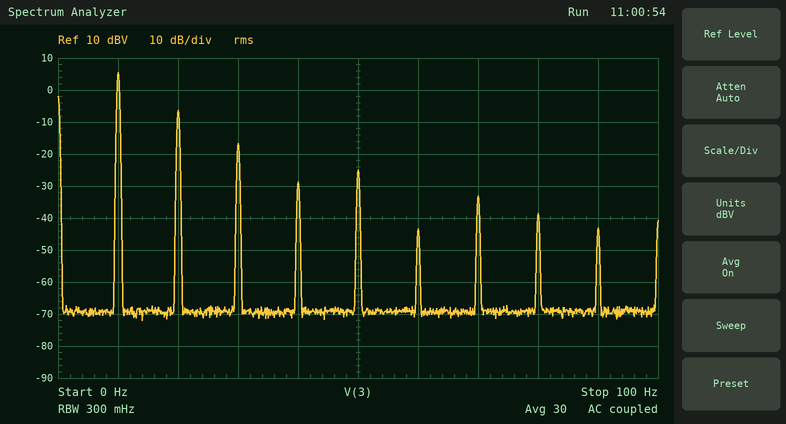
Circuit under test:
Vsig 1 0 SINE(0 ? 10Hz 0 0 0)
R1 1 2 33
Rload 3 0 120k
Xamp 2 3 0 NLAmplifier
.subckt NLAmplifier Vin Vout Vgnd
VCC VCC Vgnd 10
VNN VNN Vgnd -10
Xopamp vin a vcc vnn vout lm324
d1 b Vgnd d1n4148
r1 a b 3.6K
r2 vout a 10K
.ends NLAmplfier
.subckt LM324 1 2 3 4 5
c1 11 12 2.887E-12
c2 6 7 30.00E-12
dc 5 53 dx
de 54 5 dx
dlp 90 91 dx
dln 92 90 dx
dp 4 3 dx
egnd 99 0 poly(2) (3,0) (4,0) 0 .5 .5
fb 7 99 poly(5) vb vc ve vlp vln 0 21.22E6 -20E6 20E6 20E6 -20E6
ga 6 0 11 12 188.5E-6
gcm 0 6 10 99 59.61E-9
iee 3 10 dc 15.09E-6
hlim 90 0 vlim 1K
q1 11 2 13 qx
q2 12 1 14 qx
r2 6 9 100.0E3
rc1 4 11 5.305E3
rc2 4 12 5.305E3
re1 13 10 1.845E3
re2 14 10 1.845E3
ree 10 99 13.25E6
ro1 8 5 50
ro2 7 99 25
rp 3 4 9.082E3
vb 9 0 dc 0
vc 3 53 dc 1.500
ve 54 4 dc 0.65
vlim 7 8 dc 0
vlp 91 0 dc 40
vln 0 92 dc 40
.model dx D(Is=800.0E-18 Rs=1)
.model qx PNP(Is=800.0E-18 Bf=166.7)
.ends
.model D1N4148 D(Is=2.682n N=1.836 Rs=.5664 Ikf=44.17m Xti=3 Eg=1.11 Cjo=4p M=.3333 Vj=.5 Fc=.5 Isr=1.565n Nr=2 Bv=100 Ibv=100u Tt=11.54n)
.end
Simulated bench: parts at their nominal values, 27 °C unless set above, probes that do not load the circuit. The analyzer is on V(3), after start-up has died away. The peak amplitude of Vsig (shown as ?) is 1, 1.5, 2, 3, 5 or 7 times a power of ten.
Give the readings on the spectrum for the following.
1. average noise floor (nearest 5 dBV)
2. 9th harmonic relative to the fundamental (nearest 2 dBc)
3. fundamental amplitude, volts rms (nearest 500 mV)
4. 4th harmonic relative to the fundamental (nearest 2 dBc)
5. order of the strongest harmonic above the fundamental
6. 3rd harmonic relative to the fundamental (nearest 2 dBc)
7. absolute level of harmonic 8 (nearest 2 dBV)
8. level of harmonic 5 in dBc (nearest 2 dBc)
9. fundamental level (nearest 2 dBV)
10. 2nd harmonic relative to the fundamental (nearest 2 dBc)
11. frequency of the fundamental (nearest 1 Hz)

-70 dBV
-48 dBc
2.0 V
-34 dBc
2
-22 dBc
-38 dBV
-30 dBc
6 dBV
-12 dBc
10 Hz
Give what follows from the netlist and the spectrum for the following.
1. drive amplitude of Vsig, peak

1.5 V
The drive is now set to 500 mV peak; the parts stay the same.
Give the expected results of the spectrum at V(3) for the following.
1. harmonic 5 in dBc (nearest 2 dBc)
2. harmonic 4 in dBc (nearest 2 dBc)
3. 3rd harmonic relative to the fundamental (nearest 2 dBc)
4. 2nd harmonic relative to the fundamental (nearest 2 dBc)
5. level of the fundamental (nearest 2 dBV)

-40 dBc
-30 dBc
-24 dBc
-20 dBc
-8 dBV
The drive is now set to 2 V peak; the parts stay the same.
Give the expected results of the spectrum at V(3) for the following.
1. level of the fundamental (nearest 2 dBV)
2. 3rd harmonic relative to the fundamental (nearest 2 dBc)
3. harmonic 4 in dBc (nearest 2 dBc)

8 dBV
-24 dBc
-30 dBc
